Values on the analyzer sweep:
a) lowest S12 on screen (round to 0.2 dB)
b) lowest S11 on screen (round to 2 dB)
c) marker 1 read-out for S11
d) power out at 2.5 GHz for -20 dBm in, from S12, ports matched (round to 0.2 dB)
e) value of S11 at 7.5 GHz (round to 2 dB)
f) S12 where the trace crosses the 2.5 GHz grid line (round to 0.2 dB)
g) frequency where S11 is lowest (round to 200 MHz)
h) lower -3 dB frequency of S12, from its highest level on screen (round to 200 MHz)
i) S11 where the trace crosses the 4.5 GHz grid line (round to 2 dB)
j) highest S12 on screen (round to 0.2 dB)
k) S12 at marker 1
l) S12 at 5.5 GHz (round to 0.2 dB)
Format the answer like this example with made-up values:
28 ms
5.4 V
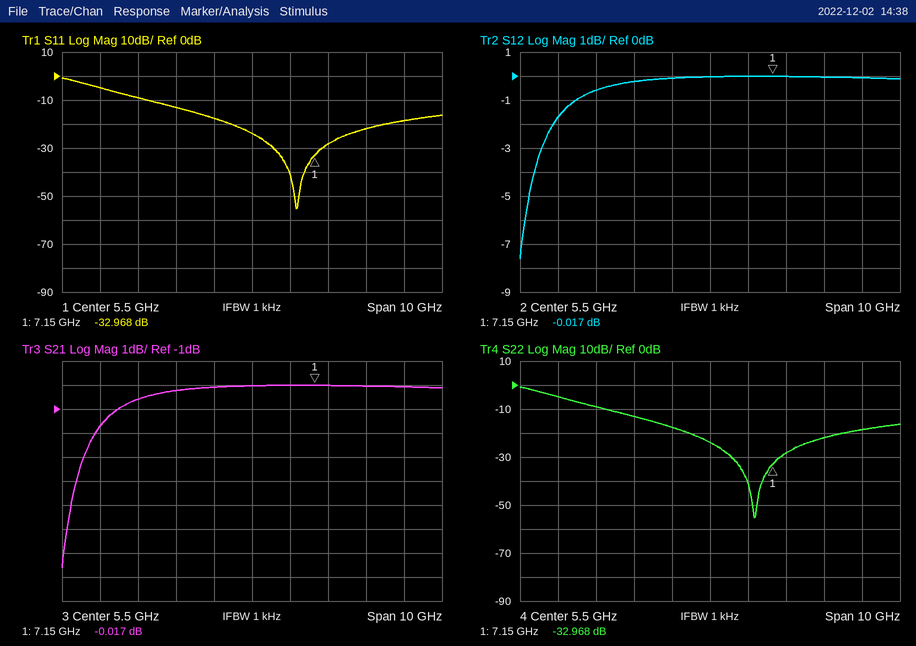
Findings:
-7.6 dB
-56 dB
-32.968 dB
-20.6 dBm
-28 dB
-0.6 dB
6.6 GHz
1.0 GHz
-18 dB
0.0 dB
-0.017 dB
0.0 dB
